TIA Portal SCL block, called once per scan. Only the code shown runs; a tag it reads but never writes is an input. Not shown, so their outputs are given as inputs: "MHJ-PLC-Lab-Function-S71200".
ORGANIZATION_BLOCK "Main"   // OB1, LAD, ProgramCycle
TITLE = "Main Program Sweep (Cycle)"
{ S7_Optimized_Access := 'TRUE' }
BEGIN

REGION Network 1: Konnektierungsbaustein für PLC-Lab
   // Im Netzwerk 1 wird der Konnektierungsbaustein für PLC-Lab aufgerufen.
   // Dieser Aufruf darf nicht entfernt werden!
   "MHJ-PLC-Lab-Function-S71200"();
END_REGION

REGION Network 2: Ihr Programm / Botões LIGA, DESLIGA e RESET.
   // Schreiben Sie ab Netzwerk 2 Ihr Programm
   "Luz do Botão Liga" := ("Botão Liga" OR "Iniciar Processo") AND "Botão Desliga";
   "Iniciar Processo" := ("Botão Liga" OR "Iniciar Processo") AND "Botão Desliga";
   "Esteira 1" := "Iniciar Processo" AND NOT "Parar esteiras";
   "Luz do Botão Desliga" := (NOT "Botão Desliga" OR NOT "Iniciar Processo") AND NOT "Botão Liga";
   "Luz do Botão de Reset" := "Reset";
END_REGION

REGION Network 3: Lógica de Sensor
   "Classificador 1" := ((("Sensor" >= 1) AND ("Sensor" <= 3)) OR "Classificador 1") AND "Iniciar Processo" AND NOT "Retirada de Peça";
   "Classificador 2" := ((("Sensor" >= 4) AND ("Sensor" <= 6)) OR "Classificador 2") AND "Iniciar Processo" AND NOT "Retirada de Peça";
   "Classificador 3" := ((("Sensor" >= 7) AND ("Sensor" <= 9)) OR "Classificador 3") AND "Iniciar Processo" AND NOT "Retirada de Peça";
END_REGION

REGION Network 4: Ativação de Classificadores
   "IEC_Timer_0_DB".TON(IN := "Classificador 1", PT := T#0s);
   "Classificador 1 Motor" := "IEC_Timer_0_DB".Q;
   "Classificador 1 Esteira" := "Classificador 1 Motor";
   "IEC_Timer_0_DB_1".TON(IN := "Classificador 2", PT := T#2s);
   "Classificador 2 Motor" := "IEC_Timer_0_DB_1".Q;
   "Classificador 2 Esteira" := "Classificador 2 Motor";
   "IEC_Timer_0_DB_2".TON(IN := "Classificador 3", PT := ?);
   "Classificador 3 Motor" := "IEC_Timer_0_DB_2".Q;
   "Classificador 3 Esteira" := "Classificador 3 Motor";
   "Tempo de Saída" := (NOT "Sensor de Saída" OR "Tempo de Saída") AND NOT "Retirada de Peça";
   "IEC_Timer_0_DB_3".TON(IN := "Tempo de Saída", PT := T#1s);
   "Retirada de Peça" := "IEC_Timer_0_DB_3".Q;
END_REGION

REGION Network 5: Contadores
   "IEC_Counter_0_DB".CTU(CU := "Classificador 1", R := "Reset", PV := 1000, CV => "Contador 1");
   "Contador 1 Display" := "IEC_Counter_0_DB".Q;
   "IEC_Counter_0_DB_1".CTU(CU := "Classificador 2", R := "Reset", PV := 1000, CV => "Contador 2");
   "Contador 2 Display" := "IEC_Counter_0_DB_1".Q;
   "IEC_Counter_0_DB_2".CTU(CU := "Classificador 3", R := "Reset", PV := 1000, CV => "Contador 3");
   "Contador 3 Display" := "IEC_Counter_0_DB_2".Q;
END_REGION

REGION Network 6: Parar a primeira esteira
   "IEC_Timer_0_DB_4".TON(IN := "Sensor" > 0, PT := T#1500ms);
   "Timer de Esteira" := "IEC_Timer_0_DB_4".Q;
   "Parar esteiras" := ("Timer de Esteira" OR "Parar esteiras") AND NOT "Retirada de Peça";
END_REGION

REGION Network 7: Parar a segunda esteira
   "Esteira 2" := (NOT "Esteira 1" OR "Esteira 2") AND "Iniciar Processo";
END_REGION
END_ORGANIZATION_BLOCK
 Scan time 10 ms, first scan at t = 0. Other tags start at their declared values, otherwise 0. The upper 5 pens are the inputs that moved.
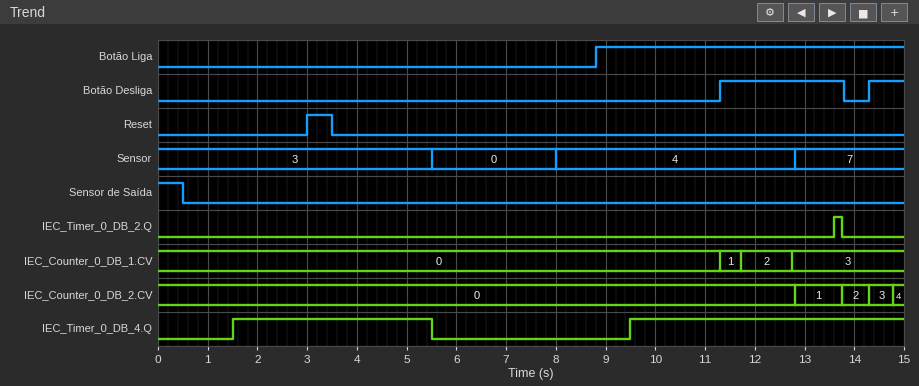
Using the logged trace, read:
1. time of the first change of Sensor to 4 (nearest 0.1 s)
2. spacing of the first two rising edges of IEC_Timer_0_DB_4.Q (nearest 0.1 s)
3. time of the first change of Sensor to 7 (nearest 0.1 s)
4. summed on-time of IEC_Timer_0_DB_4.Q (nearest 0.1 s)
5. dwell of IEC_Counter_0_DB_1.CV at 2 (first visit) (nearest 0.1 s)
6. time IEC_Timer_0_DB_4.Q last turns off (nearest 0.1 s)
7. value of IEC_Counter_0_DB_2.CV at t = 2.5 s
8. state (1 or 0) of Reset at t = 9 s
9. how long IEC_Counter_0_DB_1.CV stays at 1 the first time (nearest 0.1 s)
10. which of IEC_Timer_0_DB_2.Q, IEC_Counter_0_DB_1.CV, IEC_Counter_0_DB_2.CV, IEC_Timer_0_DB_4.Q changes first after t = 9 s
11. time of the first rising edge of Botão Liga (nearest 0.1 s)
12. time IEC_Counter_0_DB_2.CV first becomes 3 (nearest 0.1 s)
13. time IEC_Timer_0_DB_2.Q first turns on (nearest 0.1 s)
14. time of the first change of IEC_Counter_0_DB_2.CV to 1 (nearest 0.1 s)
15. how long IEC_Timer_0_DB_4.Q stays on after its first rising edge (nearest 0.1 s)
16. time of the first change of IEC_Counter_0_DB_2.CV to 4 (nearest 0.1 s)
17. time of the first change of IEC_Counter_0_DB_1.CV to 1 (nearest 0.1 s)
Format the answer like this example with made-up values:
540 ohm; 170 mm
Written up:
8.0 s; 8.0 s; 12.8 s; 9.5 s; 1.0 s; 5.5 s; 0; 0; 0.4 s; IEC_Timer_0_DB_4.Q; 8.8 s; 14.3 s; 13.6 s; 12.8 s; 4.0 s; 14.8 s; 11.3 s
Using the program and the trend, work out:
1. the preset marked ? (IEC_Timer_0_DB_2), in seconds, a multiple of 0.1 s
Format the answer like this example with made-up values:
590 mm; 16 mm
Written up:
0.8 s
